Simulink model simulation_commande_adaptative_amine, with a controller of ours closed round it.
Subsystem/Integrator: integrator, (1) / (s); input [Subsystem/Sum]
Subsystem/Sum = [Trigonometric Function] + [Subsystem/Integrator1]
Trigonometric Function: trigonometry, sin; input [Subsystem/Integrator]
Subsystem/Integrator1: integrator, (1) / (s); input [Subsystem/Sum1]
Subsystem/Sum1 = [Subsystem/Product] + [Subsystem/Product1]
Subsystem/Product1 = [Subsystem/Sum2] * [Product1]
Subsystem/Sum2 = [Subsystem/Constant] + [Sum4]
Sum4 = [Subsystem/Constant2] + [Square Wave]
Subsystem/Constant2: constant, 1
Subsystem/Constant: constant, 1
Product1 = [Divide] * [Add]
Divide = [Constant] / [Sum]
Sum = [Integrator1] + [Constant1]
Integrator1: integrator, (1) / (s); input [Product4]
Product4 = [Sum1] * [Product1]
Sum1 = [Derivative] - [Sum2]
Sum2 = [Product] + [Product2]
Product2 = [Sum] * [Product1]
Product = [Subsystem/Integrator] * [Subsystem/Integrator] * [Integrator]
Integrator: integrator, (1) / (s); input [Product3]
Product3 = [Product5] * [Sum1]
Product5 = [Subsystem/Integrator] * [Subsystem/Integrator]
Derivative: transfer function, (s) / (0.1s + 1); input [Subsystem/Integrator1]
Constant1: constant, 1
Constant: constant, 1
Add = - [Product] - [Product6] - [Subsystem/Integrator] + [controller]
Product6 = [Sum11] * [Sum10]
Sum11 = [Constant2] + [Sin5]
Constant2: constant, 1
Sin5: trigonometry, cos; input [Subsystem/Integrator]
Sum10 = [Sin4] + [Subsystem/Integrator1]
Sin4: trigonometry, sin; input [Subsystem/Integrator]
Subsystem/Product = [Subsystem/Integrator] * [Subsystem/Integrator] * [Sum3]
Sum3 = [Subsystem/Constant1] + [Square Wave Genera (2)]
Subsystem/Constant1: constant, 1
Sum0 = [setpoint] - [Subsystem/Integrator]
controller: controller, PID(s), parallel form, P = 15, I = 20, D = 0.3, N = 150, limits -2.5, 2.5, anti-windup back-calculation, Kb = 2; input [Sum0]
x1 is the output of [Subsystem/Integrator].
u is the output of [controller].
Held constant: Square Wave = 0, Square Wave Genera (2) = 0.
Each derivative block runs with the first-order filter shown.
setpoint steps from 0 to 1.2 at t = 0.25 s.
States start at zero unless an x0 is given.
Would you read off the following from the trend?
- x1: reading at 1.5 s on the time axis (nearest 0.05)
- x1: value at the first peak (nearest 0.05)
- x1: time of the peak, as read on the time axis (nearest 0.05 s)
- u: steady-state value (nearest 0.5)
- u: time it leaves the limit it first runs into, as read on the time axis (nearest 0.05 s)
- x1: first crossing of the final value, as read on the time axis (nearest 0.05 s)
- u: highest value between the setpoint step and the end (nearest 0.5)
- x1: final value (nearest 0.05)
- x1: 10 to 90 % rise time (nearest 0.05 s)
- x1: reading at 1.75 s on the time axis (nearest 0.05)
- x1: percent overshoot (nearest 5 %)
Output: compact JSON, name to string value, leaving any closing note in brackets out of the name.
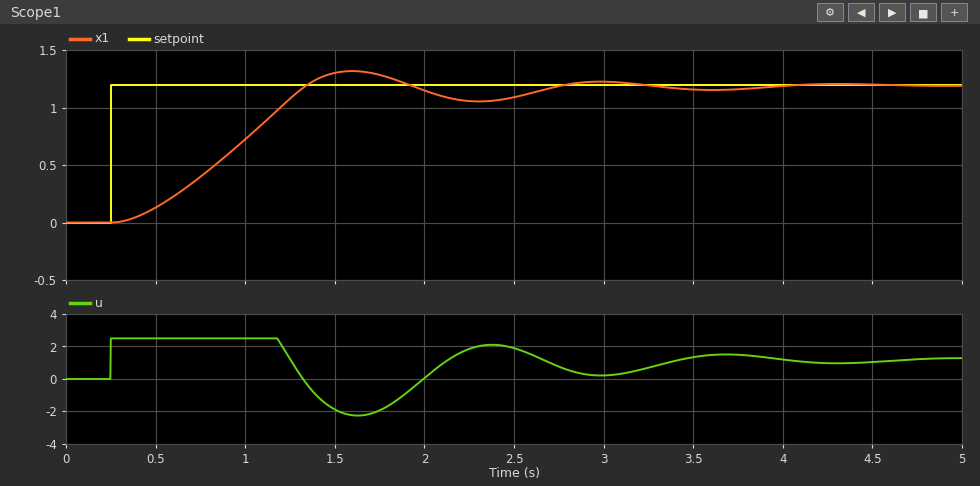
{"x1: reading at 1.5 s on the time axis": "1.30", "x1: value at the first peak": "1.30", "x1: time of the peak, as read on the time axis": "1.60 s", "u: steady-state value": "1.0", "u: time it leaves the limit it first runs into, as read on the time axis": "1.20 s", "x1: first crossing of the final value, as read on the time axis": "1.35 s", "u: highest value between the setpoint step and the end": "2.5", "x1: final value": "1.20", "x1: 10 to 90 % rise time": "0.75 s", "x1: reading at 1.75 s on the time axis": "1.30", "x1: percent overshoot": "10 %"}
